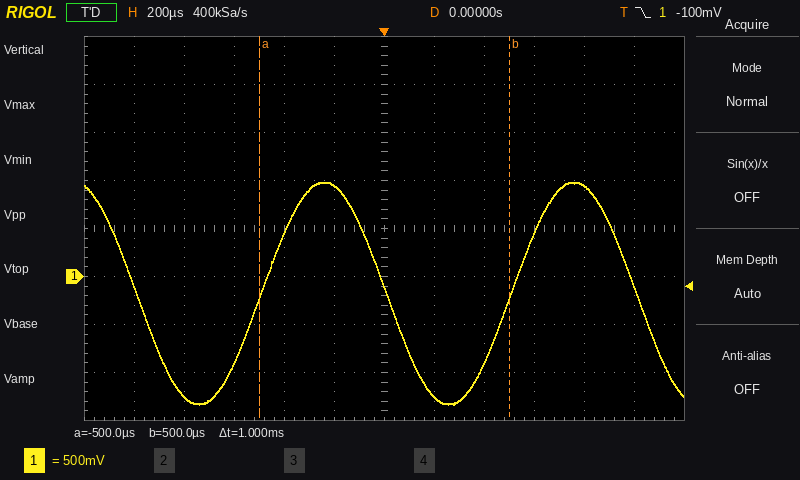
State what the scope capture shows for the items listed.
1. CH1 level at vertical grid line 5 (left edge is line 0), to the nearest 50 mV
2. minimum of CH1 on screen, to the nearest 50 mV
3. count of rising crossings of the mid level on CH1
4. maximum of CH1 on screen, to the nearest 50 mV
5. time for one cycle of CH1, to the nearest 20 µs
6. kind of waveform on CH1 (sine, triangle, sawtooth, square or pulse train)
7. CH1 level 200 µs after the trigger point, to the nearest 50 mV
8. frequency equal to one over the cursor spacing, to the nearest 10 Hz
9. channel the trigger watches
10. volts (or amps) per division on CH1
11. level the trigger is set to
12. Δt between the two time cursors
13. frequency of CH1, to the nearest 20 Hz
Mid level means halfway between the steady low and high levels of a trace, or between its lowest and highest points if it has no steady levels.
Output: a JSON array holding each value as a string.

["950 mV", "-1.35 V", "2", "1.00 V", "1.00 ms", "sine", "-1.25 V", "1.00 kHz", "CH1", "500 mV", "-100 mV", "1 ms", "1.00 kHz"]
